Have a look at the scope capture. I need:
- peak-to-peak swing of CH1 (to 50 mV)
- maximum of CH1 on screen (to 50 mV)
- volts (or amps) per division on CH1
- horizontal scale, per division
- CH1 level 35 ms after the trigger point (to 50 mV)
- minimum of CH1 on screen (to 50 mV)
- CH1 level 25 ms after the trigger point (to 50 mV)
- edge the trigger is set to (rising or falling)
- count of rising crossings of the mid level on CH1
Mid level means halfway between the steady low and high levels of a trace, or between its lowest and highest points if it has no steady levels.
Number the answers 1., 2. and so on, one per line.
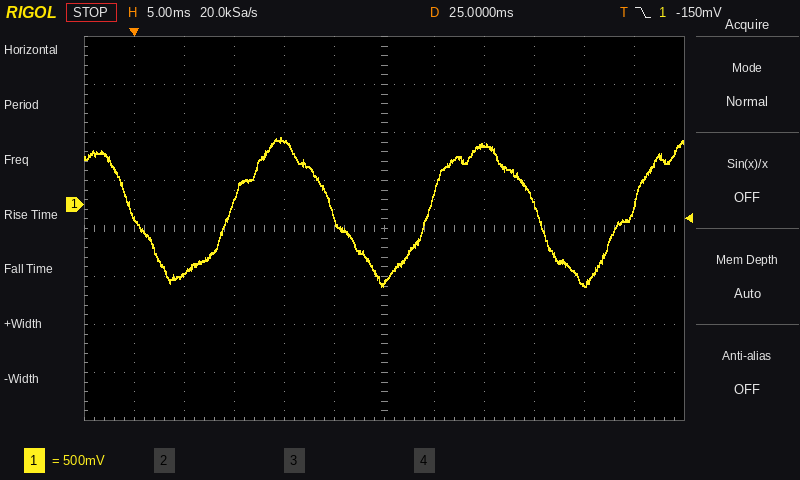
1. 1.55 V
2. 700 mV
3. 500 mV
4. 5 ms
5. 600 mV
6. -850 mV
7. -800 mV
8. falling
9. 3
